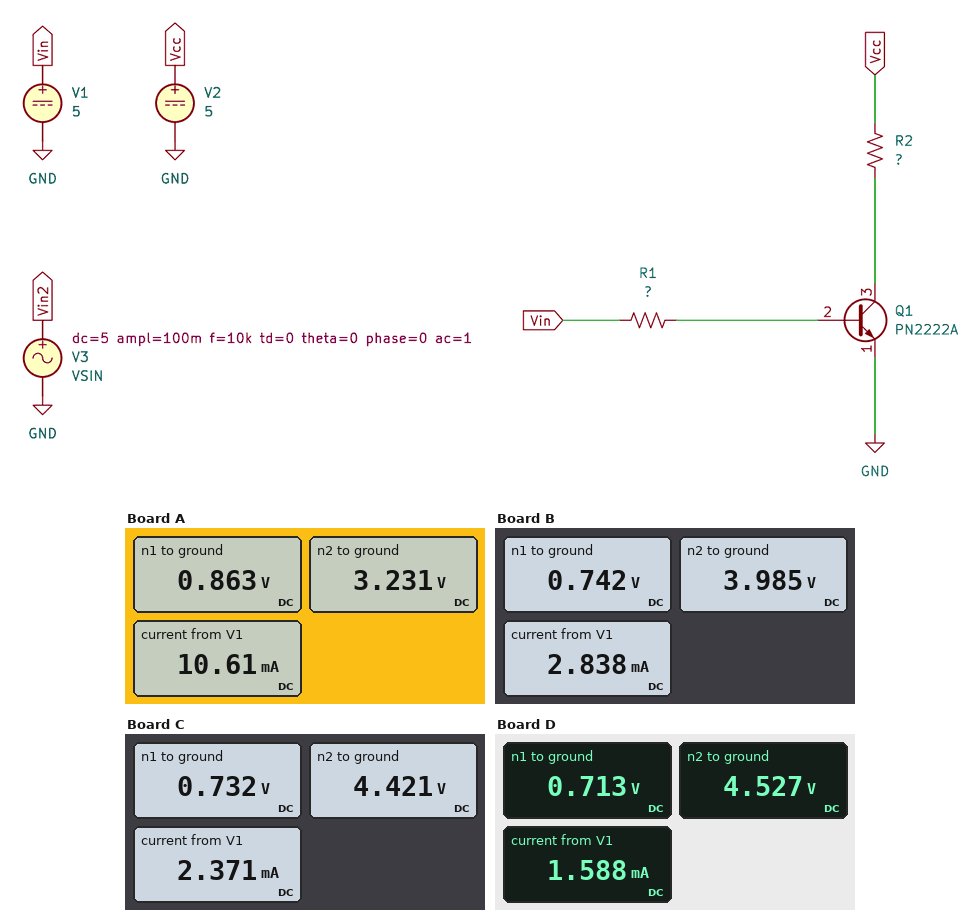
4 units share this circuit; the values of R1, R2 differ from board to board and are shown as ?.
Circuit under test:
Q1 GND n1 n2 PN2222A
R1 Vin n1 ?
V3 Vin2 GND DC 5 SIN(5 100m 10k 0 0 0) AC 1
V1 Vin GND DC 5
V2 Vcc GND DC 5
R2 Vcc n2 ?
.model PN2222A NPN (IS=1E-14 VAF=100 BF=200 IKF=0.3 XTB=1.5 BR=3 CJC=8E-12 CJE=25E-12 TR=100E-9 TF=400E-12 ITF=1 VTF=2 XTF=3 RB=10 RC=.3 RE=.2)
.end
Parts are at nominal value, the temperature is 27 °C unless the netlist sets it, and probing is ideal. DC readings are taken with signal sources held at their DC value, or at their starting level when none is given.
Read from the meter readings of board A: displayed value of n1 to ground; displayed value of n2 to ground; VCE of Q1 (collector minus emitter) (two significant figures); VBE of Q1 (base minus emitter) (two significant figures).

0.863 V
3.231 V
-3.2 V
-2.4 V
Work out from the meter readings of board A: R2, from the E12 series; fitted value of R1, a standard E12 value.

56 Ω
390 Ω
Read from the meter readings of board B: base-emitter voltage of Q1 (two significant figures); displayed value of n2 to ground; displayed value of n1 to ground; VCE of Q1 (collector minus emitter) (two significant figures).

-3.2 V
3.985 V
0.742 V
-4.0 V
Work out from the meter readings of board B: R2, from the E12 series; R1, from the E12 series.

120 Ω
1.5 kΩ
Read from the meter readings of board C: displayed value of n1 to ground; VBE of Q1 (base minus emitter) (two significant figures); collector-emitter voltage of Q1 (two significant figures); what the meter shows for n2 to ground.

0.732 V
-3.7 V
-4.4 V
4.421 V
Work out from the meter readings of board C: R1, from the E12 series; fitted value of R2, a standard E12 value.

1.8 kΩ
82 Ω
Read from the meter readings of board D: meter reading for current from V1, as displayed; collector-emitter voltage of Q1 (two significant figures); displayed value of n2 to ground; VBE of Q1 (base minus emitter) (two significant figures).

1.588 mA
-4.5 V
4.527 V
-3.8 V
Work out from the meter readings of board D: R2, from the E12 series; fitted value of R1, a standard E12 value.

100 Ω
2.7 kΩ
